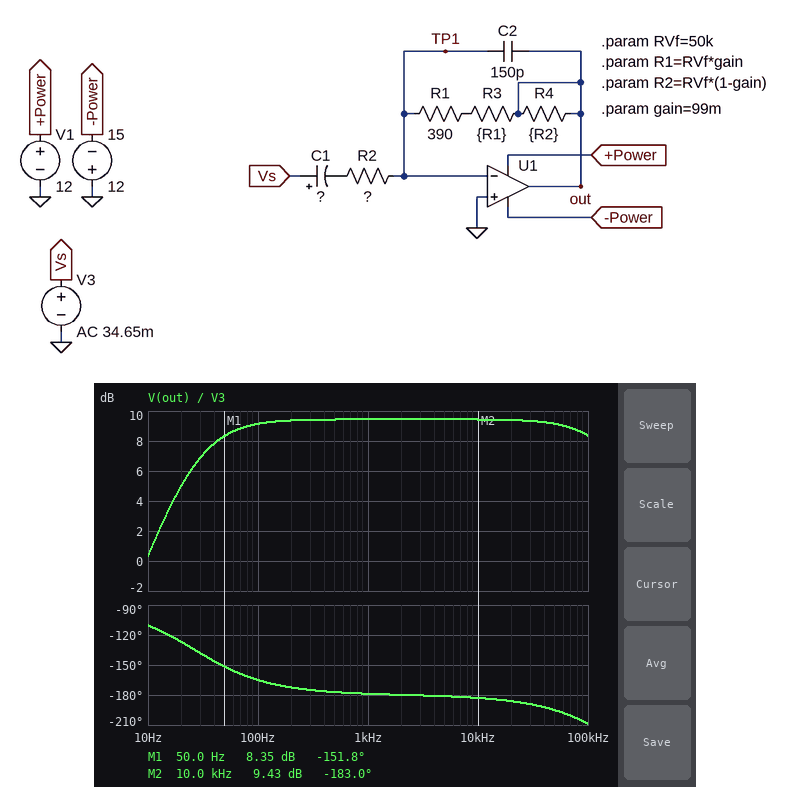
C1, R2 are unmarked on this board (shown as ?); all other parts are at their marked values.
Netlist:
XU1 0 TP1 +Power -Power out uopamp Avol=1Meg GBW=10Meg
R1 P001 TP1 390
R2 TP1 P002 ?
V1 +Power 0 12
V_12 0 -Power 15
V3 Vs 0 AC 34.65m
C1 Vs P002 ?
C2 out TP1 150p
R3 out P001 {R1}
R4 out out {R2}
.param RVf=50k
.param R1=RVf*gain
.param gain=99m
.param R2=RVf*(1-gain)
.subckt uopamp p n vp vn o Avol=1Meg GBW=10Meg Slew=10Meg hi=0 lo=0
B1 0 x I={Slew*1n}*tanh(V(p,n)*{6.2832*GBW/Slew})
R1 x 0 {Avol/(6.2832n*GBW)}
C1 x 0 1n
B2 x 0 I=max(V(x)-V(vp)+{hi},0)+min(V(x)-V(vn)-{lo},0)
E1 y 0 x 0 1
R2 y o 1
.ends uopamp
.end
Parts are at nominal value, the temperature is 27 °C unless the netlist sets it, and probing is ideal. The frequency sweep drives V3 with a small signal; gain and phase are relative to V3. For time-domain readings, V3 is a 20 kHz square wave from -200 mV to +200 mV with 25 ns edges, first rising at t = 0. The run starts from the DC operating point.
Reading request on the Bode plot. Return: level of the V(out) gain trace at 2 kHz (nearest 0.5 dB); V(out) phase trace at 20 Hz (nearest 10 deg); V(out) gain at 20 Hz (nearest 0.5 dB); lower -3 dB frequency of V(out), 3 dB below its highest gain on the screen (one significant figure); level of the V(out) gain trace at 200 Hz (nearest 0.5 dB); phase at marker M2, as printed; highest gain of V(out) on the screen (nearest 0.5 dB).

9.5 dB
-130 deg
5.0 dB
30 Hz
9.5 dB
-183.0 deg
9.5 dB
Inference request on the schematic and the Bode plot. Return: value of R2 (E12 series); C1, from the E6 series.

1.8 kΩ
3.3 µF
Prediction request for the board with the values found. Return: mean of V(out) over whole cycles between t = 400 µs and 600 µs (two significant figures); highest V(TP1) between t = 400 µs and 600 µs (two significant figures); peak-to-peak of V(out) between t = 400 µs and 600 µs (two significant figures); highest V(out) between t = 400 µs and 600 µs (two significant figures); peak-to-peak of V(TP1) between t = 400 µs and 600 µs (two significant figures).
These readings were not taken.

-540 mV
21 mV
1.2 V
57 mV
42 mV
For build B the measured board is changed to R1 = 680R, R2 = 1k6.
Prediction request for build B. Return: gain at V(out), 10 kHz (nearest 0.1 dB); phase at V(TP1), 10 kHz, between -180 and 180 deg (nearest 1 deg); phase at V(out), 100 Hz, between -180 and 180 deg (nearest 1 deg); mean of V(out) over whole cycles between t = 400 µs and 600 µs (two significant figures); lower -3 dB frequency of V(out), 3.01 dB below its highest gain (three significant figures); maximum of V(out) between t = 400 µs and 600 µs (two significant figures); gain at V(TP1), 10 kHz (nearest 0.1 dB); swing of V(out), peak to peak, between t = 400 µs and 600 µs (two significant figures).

10.9 dB
87 deg
-163 deg
-640 mV
30.1 Hz
76 mV
-49.1 dB
1.4 V
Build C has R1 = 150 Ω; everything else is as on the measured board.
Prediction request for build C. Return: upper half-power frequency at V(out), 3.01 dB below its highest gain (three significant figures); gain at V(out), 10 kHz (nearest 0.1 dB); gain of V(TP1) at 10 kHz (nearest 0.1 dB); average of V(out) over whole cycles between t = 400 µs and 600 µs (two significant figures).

196 kHz
9.0 dB
-51.0 dB
-520 mV
